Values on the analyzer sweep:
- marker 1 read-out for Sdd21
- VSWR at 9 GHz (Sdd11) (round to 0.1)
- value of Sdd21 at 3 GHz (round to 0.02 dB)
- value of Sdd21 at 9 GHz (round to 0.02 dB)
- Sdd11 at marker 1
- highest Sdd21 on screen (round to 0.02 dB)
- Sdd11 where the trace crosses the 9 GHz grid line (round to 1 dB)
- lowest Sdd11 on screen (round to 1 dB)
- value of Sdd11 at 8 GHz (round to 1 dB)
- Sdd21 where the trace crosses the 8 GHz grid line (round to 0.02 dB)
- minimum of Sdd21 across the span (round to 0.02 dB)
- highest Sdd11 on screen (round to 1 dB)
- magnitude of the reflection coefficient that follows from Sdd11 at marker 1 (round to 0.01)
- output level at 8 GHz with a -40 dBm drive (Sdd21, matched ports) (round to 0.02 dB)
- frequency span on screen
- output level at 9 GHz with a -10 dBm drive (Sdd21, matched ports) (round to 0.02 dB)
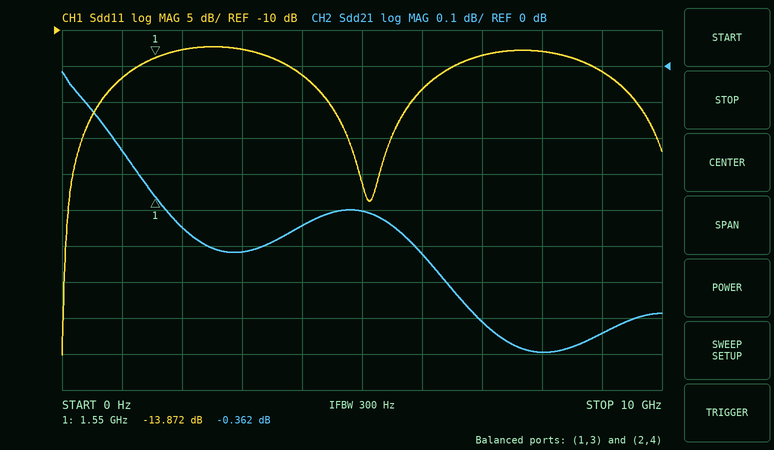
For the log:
-0.362 dB
1.4
-0.52 dB
-0.74 dB
-13.872 dB
-0.02 dB
-16 dB
-55 dB
-13 dB
-0.80 dB
-0.80 dB
-12 dB
0.20
-40.80 dBm
10 GHz
-10.74 dBm
